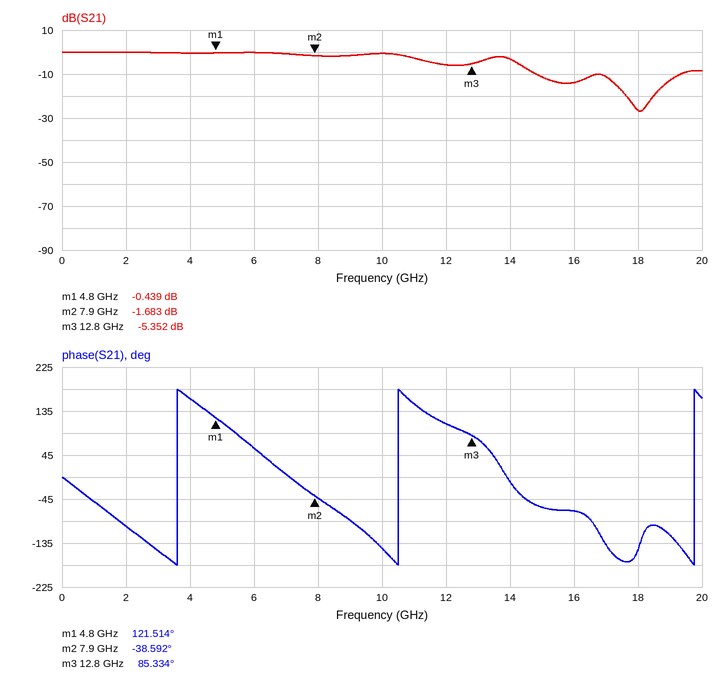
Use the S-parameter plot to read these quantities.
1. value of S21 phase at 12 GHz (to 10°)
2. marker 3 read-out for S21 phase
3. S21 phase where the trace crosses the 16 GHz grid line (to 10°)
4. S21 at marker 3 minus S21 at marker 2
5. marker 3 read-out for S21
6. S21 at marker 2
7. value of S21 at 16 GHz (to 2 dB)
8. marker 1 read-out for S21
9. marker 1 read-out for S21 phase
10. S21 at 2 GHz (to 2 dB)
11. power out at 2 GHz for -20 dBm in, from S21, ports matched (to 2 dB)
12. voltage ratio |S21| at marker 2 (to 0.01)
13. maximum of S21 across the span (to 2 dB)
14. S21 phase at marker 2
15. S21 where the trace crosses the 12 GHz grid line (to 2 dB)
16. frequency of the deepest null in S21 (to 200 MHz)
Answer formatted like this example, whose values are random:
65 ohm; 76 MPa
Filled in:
110°; 85.334°; -70°; -3.669 dB; -5.352 dB; -1.683 dB; -14 dB; -0.439 dB; 121.514°; 0 dB; -20 dBm; 0.82; 0 dB; -38.592°; -6 dB; 18.0 GHz
